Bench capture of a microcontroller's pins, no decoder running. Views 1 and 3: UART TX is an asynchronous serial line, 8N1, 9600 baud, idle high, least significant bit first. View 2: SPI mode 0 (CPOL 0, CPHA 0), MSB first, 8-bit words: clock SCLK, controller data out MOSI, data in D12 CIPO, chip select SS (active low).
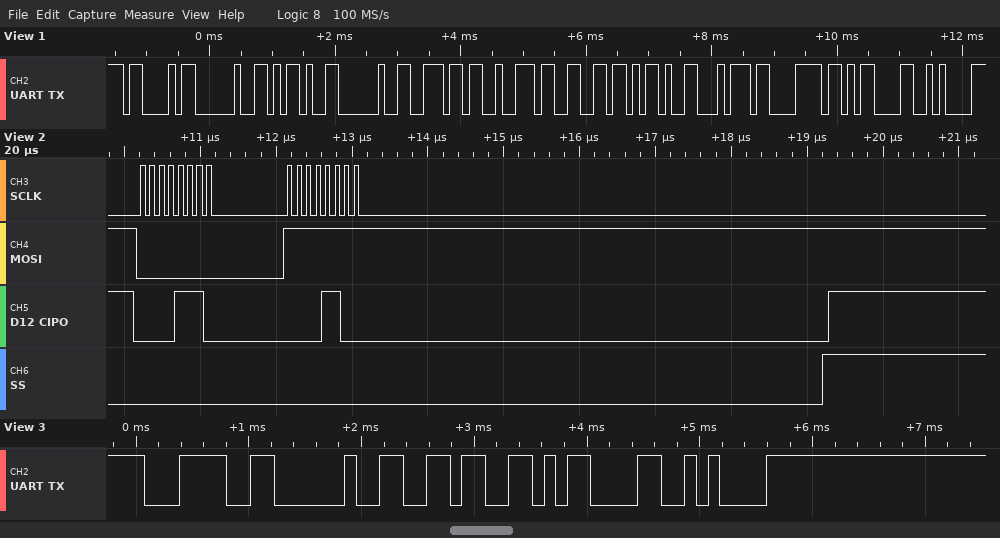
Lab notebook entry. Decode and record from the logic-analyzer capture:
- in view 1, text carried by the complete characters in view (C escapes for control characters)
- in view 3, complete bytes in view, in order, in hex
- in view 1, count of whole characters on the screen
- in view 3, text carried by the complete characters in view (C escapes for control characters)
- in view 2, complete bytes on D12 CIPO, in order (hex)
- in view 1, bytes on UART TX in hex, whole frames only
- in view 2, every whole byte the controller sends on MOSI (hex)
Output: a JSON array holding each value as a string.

["\"C - nrf-tx\\r\\n\"", "0x3C 0x20 0x36 0x0D 0x0A", "12", "\"< 6\\r\\n\"", "0E 0C", "0x43 0x20 0x2D 0x20 0x6E 0x72 0x66 0x2D 0x74 0x78 0x0D 0x0A", "00 FF"]
